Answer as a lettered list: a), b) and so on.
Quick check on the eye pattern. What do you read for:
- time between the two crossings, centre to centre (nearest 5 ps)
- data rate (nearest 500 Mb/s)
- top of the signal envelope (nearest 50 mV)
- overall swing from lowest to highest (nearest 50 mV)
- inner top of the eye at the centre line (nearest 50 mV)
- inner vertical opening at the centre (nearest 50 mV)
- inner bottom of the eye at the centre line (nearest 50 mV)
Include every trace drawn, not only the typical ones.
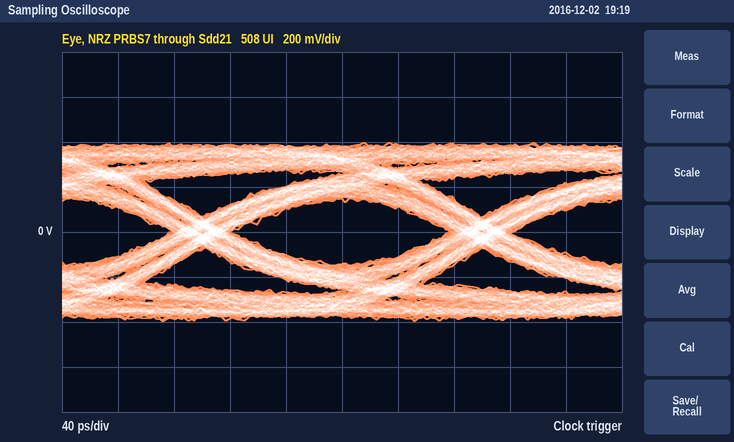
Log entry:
a) 200 ps
b) 5.0 Gb/s
c) 400 mV
d) 800 mV
e) 150 mV
f) 300 mV
g) -150 mV
